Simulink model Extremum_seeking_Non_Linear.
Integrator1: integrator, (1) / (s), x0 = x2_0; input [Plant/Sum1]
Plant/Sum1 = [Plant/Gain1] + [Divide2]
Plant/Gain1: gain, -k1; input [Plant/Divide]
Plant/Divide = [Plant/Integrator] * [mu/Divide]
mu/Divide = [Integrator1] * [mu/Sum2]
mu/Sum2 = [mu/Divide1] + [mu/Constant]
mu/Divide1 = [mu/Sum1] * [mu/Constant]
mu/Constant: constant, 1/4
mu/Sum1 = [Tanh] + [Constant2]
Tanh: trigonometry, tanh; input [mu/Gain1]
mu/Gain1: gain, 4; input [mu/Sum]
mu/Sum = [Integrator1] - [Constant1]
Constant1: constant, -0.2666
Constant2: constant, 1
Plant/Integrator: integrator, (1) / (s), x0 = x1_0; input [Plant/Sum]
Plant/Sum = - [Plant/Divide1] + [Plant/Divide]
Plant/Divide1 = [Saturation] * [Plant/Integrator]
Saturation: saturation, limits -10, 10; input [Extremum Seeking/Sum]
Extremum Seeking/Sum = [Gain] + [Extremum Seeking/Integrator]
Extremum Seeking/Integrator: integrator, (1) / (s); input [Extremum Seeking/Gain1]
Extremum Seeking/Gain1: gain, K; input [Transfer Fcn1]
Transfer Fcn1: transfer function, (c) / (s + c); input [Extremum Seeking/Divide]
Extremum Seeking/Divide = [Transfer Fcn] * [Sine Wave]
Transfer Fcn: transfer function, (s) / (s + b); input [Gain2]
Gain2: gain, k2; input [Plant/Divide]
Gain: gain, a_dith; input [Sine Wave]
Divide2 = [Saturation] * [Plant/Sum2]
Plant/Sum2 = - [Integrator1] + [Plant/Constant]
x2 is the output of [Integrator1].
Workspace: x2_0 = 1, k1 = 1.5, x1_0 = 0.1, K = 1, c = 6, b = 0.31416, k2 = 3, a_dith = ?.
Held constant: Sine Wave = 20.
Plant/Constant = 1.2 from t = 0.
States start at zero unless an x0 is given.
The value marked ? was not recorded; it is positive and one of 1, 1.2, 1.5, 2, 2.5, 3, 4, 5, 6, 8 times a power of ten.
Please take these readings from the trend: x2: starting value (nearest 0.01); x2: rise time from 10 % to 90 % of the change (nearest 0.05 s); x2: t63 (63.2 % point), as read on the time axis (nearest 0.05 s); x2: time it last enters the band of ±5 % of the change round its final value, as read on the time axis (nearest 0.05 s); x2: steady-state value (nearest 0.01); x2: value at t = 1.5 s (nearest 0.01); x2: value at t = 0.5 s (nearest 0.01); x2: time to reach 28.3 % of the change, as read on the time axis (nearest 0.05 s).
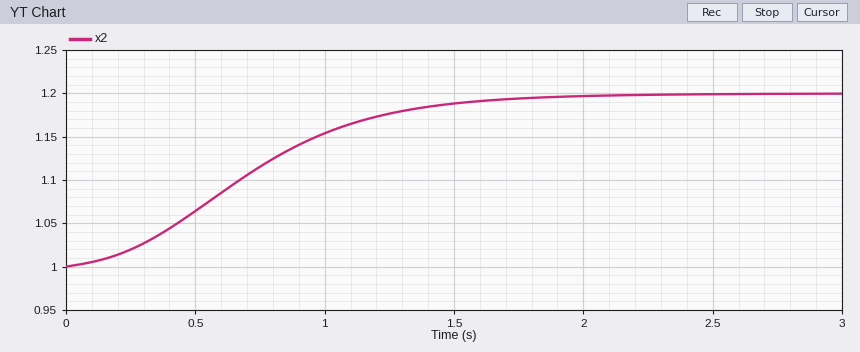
1.00
1.05 s
0.80 s
1.55 s
1.20
1.19
1.06
0.45 s
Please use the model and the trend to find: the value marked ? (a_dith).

0.04
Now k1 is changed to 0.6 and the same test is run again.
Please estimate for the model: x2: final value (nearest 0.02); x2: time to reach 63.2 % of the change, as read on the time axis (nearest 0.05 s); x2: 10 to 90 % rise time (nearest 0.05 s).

1.20
0.70 s
1.00 s
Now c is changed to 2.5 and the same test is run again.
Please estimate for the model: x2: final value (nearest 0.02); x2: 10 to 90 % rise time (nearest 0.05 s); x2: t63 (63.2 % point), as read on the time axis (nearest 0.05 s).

1.20
1.15 s
0.95 s
